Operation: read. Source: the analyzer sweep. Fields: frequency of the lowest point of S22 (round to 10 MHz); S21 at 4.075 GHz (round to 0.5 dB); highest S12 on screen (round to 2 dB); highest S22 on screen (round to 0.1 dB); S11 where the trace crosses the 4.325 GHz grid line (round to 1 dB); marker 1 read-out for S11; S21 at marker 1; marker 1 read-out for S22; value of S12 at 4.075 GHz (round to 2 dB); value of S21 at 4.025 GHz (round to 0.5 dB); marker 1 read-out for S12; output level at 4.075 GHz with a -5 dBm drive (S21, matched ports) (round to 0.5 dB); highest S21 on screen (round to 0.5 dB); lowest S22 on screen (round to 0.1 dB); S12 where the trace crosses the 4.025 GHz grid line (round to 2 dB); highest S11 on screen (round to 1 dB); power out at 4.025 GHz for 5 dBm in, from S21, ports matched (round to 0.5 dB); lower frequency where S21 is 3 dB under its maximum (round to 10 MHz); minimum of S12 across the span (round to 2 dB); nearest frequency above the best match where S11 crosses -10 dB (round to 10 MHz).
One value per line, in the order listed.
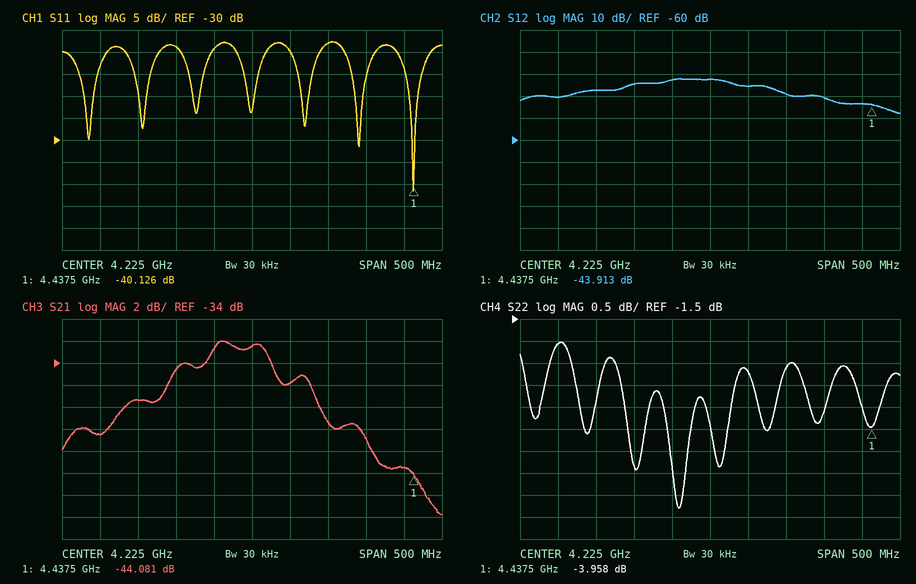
4.18 GHz
-37.5 dB
-32 dB
-2.0 dB
-8 dB
-40.126 dB
-44.081 dB
-3.958 dB
-38 dB
-40.5 dB
-43.913 dB
-42.5 dBm
-32.0 dB
-5.8 dB
-40 dB
-8 dB
-35.5 dBm
4.12 GHz
-48 dB
4.46 GHz
